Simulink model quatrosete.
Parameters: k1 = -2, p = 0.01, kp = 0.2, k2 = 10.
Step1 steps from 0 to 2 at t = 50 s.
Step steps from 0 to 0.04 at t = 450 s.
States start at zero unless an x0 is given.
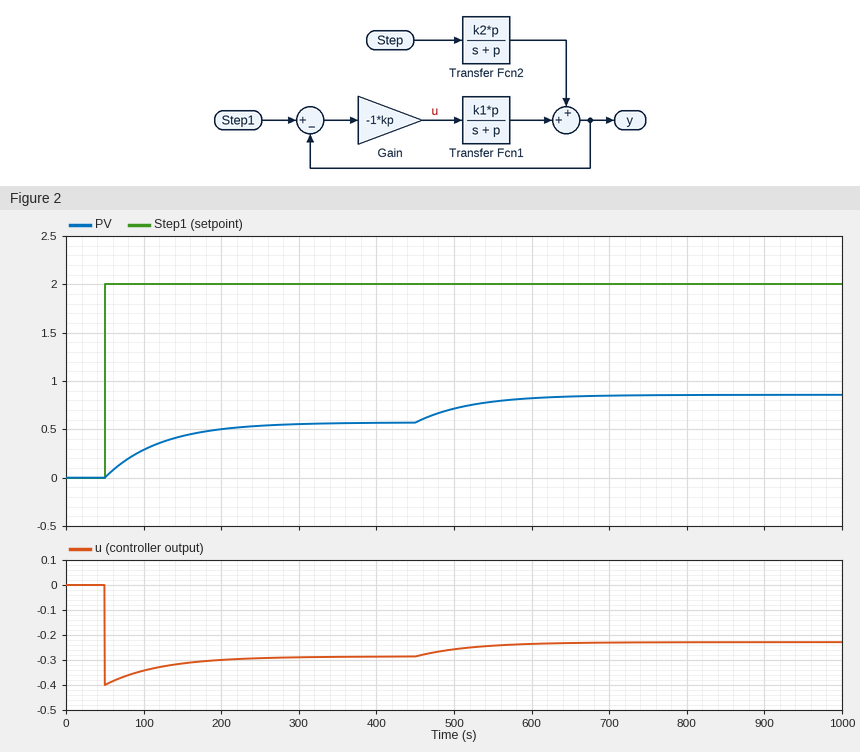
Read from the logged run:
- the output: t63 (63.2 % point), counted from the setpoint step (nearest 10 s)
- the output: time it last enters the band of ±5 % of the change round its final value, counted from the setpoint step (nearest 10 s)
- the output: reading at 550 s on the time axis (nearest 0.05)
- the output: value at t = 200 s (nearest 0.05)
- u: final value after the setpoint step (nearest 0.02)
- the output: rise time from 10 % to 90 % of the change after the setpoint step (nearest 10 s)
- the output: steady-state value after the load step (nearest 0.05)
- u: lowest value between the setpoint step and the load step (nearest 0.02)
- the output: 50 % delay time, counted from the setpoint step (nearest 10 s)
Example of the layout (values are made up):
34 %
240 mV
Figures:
70 s
210 s
0.80
0.50
-0.28
160 s
0.85
-0.40
50 s
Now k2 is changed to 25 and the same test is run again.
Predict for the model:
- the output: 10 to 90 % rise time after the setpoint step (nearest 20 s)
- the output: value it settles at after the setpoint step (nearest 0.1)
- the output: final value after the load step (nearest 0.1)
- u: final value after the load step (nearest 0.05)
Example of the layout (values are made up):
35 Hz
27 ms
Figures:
160 s
0.6
1.3
-0.15
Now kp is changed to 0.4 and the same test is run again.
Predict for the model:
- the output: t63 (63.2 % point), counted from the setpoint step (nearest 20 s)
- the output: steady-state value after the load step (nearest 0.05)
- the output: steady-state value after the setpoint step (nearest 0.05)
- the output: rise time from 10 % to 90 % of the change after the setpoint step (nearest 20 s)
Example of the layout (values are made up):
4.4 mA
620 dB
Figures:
60 s
1.10
0.90
120 s
